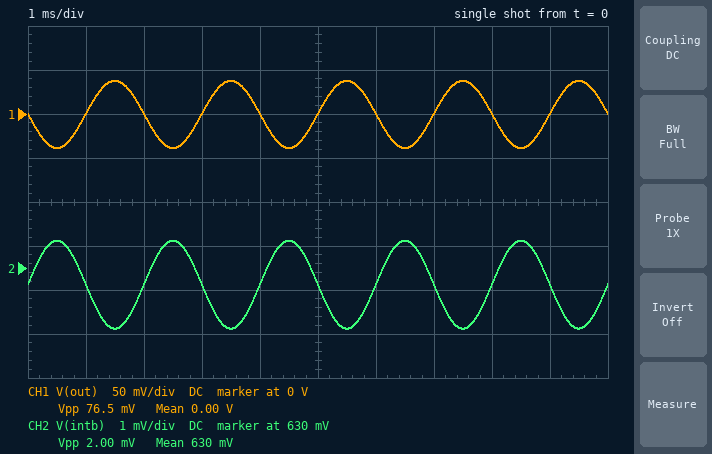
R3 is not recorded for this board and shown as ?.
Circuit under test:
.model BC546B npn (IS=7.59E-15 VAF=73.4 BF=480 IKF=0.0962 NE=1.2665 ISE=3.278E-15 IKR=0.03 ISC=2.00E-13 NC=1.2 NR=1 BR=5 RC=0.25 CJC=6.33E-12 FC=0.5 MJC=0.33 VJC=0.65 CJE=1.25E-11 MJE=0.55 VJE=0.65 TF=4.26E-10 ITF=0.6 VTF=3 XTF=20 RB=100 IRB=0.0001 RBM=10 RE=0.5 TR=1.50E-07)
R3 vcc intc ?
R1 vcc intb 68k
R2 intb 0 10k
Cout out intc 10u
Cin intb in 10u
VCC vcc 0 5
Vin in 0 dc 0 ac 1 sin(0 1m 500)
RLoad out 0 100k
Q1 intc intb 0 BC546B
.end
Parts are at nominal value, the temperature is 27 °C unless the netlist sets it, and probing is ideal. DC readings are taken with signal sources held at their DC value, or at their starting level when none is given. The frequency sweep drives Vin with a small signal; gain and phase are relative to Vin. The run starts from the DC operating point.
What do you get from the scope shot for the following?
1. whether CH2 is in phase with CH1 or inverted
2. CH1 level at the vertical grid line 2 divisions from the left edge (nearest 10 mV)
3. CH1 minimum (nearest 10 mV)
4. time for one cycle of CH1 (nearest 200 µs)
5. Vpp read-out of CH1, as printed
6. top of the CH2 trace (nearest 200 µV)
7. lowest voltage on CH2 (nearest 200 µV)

inverted
0 V
-40 mV
2.0 ms
76.5 mV
630.6 mV
628.6 mV
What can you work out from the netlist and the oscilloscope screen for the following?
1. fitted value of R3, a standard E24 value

3.6 kΩ
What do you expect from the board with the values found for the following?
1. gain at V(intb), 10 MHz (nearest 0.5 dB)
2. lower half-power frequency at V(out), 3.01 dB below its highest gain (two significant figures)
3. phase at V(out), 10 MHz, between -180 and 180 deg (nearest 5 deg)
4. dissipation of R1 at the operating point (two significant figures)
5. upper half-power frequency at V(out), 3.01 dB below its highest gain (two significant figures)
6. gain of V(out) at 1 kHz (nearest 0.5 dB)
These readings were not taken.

0 dB
2.5 Hz
115 deg
280 µW
5.9 MHz
31.5 dB
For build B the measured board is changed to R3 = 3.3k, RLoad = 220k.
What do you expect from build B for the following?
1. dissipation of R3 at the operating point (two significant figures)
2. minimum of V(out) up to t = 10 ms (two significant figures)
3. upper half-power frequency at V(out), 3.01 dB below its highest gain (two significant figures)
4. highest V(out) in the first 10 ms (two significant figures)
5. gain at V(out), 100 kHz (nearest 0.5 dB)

280 µW
-36 mV
6.3 MHz
35 mV
31.0 dB
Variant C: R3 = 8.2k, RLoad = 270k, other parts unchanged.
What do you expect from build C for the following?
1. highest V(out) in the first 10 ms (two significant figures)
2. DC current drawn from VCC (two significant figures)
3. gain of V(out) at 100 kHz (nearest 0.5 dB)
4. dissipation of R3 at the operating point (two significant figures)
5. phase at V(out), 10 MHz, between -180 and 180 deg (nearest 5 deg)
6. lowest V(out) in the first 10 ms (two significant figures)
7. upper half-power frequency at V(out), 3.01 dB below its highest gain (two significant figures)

84 mV
350 µA
38.5 dB
680 µW
95 deg
-86 mV
2.4 MHz
